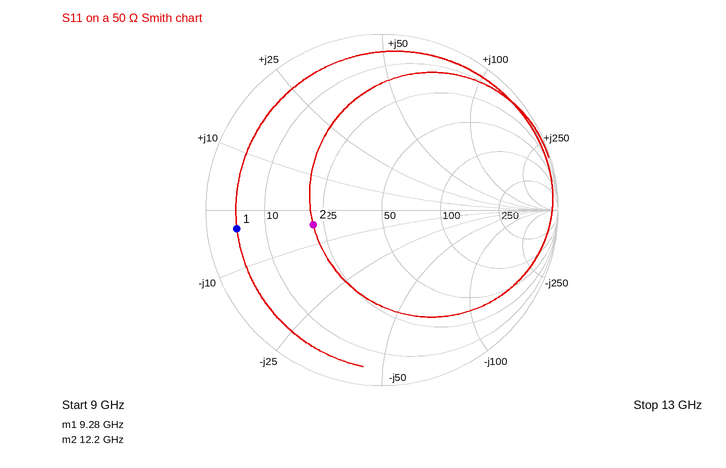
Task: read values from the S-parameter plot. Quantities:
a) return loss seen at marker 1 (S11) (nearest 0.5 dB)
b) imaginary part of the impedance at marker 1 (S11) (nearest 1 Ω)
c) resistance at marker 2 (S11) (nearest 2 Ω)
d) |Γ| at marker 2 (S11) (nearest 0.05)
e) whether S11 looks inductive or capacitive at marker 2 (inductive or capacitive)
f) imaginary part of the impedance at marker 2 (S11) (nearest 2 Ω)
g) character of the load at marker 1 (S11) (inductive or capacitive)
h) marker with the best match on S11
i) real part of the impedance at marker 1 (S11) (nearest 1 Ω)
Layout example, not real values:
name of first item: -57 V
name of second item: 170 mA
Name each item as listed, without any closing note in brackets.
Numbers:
return loss seen at marker 1 (S11): 1.5 dB
imaginary part of the impedance at marker 1 (S11): -3 Ω
resistance at marker 2 (S11): 22 Ω
|Γ| at marker 2 (S11): 0.40
whether S11 looks inductive or capacitive at marker 2: capacitive
imaginary part of the impedance at marker 2 (S11): -4 Ω
character of the load at marker 1 (S11): capacitive
marker with the best match on S11: marker 2
real part of the impedance at marker 1 (S11): 5 Ω
